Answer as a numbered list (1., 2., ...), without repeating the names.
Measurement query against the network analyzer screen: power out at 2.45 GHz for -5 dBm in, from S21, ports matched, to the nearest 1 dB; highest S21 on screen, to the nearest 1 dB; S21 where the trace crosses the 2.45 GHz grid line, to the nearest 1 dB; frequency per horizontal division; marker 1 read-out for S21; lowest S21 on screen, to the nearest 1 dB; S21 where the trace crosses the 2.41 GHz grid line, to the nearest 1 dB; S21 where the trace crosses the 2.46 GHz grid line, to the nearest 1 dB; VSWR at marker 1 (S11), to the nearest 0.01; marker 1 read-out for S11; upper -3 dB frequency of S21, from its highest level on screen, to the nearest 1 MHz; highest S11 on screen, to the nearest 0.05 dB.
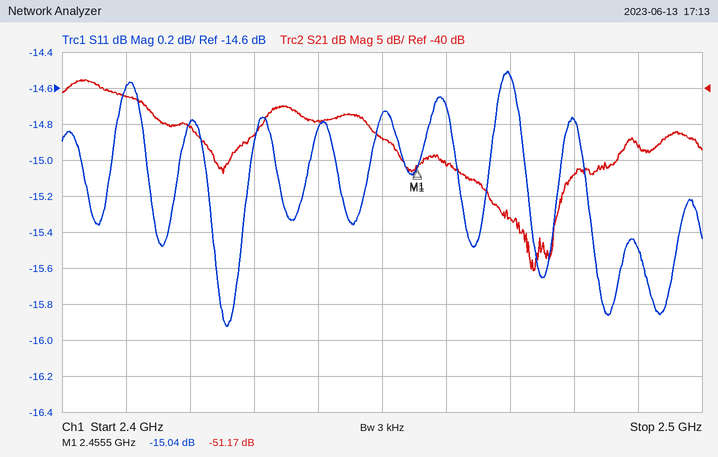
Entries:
1. -52 dBm
2. -39 dB
3. -47 dB
4. 10 MHz
5. -51.17 dB
6. -65 dB
7. -41 dB
8. -51 dB
9. 1.43
10. -15.04 dB
11. 2.412 GHz
12. -14.50 dB
